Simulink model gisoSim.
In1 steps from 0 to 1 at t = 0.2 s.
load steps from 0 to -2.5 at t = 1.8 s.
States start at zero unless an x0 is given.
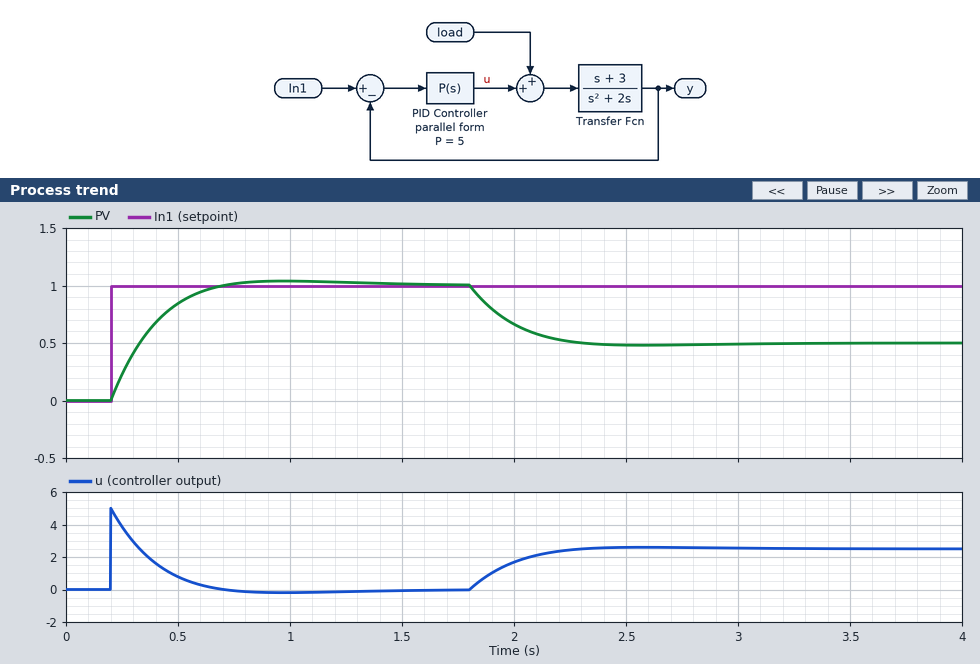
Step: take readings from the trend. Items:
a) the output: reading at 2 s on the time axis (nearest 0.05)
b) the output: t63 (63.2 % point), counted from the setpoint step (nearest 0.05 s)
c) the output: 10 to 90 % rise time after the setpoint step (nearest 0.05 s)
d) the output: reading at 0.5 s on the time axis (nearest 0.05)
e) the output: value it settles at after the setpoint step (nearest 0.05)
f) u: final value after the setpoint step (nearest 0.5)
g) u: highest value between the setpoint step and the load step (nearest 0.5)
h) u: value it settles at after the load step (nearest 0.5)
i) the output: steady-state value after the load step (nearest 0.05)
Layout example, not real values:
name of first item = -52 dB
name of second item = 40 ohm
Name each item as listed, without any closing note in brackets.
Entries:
the output: reading at 2 s on the time axis = 0.65
the output: t63 (63.2 % point), counted from the setpoint step = 0.20 s
the output: 10 to 90 % rise time after the setpoint step = 0.35 s
the output: reading at 0.5 s on the time axis = 0.85
the output: value it settles at after the setpoint step = 1.00
u: final value after the setpoint step = 0.0
u: highest value between the setpoint step and the load step = 5.0
u: value it settles at after the load step = 2.5
the output: steady-state value after the load step = 0.50
